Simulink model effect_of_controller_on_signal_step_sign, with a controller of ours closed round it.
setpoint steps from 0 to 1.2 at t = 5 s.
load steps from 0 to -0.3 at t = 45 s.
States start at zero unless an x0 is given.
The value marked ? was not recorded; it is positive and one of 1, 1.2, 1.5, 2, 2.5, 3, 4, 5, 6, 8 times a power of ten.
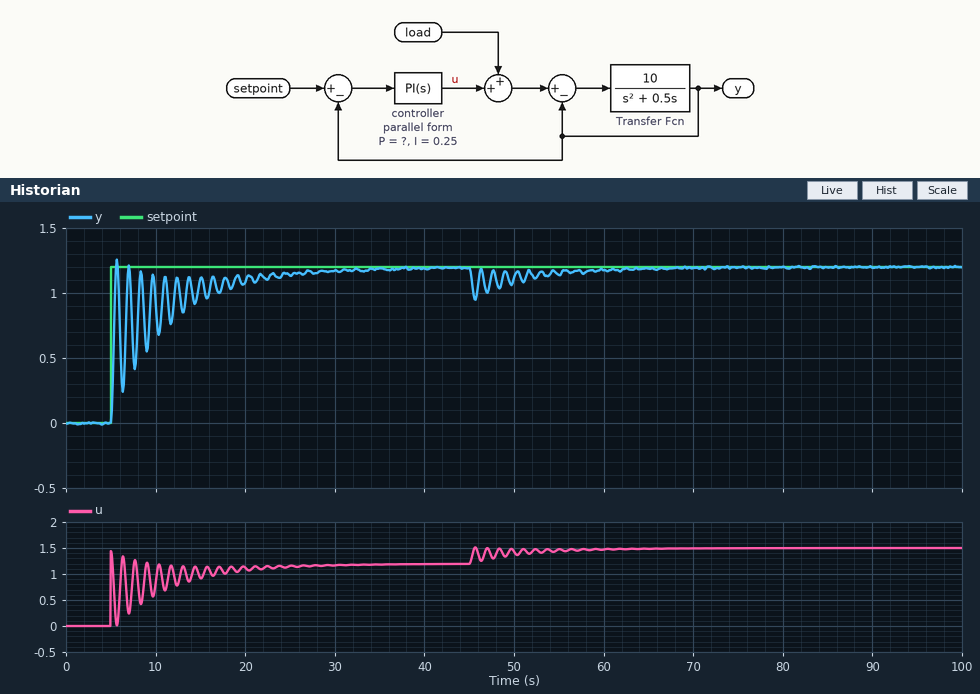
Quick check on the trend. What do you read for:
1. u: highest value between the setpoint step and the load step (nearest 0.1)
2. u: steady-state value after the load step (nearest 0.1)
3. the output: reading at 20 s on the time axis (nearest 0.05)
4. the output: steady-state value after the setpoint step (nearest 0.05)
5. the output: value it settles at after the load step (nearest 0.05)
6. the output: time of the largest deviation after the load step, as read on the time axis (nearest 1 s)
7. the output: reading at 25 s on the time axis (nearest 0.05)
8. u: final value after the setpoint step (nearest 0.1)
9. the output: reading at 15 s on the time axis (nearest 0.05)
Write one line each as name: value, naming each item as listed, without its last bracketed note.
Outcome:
u: highest value between the setpoint step and the load step: 1.4
u: steady-state value after the load step: 1.5
the output: reading at 20 s on the time axis: 1.10
the output: steady-state value after the setpoint step: 1.20
the output: value it settles at after the load step: 1.20
the output: time of the largest deviation after the load step, as read on the time axis: 46 s
the output: reading at 25 s on the time axis: 1.15
u: final value after the setpoint step: 1.2
the output: reading at 15 s on the time axis: 1.10
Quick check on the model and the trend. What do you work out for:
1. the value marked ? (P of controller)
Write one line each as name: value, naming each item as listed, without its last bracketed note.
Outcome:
the value marked ?: 1.2
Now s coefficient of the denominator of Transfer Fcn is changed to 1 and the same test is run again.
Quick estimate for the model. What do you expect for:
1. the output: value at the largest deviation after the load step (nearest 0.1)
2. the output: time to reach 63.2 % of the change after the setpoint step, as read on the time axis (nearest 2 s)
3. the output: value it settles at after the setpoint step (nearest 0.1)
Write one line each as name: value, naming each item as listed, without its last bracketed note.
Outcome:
the output: value at the largest deviation after the load step: 1.0
the output: time to reach 63.2 % of the change after the setpoint step, as read on the time axis: 6 s
the output: value it settles at after the setpoint step: 1.2
